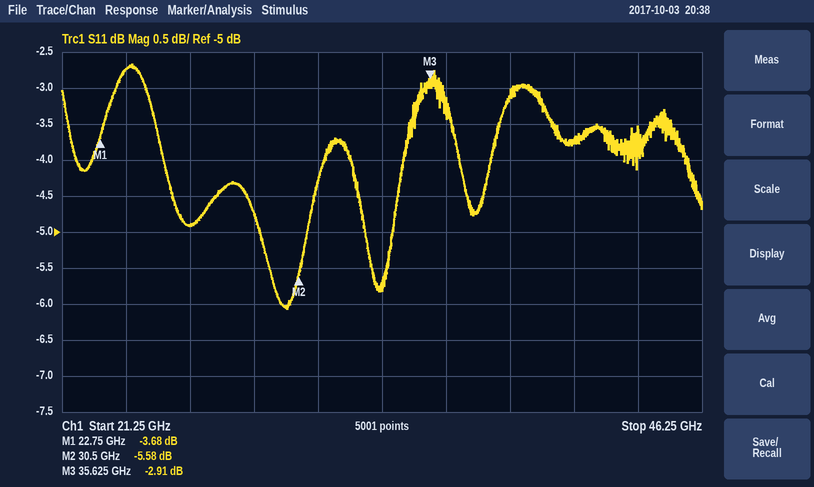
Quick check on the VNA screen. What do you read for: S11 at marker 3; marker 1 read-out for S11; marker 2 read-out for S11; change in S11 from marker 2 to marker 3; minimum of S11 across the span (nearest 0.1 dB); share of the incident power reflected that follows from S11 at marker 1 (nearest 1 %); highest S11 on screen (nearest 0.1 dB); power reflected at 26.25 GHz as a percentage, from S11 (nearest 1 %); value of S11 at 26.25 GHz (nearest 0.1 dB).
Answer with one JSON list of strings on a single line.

["-2.91 dB", "-3.68 dB", "-5.58 dB", "2.67 dB", "-6.1 dB", "43 %", "-2.7 dB", "32 %", "-4.9 dB"]
